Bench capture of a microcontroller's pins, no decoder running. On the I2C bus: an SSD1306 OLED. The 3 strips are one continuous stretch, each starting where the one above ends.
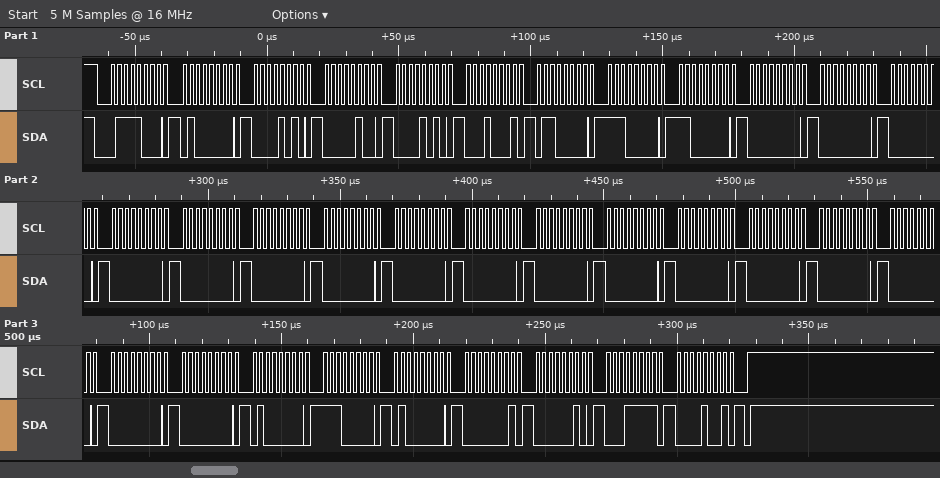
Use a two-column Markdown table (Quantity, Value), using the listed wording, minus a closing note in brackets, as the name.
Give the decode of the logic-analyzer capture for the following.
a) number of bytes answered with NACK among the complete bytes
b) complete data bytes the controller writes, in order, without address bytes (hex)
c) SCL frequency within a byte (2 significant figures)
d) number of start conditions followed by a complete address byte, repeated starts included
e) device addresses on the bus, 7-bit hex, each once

| Quantity | Value |
|---|---|
| number of bytes answered with NACK among the complete bytes | 0 |
| complete data bytes the controller writes, in order, without address bytes | 40 0A 04 0A 11 60 E0 C0 00 00 00 00 00 00 00 00 00 00 00 00 00 00 00 00 00 40 E0 40 01 02 1F 09 |
| SCL frequency within a byte | 400 kHz |
| number of start conditions followed by a complete address byte, repeated starts included | 1 |
| device addresses on the bus, 7-bit hex, each once | 0x3C |
